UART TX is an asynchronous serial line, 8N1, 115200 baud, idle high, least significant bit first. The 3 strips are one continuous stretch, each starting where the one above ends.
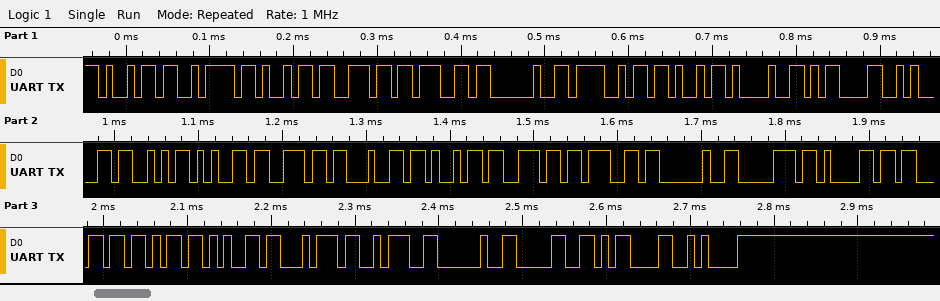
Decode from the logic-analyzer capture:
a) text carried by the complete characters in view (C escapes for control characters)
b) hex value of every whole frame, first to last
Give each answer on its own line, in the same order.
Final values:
"izing OK!\r\nSending packet: 0\r\n"
69 7A 69 6E 67 20 4F 4B 21 0D 0A 53 65 6E 64 69 6E 67 20 70 61 63 6B 65 74 3A 20 30 0D 0A
